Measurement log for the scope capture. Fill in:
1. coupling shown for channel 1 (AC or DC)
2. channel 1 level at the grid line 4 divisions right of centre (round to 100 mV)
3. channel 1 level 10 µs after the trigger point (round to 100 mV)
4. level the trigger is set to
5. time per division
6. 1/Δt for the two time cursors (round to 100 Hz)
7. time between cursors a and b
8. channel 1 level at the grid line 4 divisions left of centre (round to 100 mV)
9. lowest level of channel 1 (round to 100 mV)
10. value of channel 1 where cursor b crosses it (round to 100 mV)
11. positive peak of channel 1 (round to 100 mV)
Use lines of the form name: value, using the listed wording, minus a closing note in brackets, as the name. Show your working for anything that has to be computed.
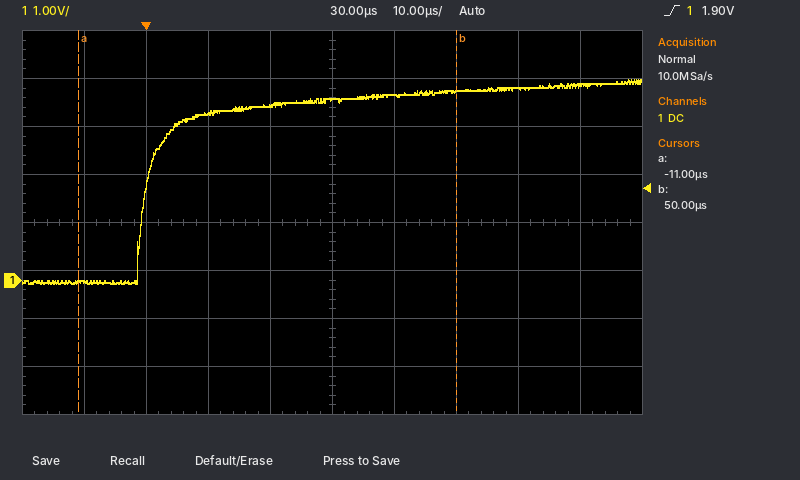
coupling shown for channel 1: DC
channel 1 level at the grid line 4 divisions right of centre: 4.1 V
channel 1 level 10 µs after the trigger point: 3.5 V
level the trigger is set to: 1.90 V
time per division: 10 µs
1/Δt for the two time cursors: 1 / 61 µs ≈ 16.4 kHz
time between cursors a and b: 50 µs − (-11 µs) = 61 µs
channel 1 level at the grid line 4 divisions left of centre: 0.0 V
lowest level of channel 1: -100 mV
value of channel 1 where cursor b crosses it: 3.9 V
positive peak of channel 1: 4.2 V
